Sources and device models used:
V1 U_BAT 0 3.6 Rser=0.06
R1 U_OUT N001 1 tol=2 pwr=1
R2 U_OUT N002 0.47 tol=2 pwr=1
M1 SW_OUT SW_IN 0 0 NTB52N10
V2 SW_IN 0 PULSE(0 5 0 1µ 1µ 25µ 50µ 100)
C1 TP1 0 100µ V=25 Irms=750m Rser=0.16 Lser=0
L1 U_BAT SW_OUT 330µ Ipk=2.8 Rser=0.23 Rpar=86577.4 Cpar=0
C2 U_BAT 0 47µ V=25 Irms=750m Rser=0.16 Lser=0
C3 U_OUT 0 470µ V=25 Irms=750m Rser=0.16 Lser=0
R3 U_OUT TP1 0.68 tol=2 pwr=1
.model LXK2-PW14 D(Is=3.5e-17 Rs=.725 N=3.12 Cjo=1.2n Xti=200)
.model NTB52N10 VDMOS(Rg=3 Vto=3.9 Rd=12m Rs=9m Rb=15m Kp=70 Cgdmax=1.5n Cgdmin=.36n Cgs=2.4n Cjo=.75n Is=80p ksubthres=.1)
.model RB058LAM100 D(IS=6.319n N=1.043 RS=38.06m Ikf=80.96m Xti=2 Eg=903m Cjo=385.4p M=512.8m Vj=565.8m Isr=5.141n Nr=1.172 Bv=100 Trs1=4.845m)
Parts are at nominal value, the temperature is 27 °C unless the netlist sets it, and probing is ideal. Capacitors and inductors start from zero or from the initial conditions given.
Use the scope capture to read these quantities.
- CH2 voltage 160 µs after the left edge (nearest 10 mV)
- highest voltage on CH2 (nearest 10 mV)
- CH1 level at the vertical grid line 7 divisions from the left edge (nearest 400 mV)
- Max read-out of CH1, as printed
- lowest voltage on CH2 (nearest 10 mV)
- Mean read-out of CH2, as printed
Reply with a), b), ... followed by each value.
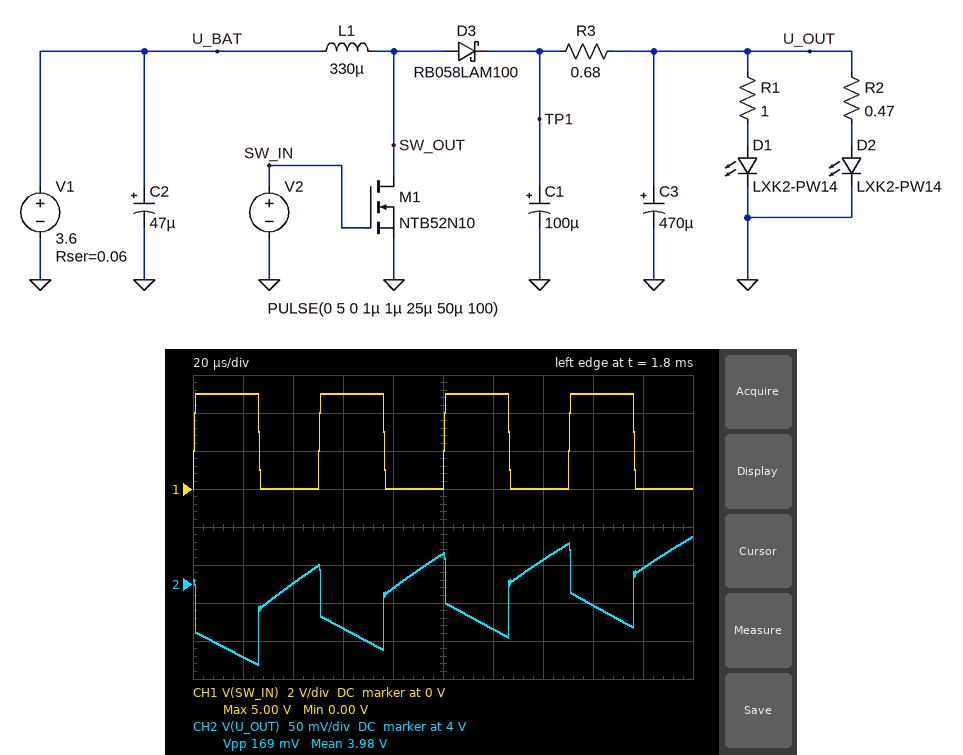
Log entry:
a) 3.97 V
b) 4.06 V
c) 0 V
d) 5.00 V
e) 3.89 V
f) 3.98 V
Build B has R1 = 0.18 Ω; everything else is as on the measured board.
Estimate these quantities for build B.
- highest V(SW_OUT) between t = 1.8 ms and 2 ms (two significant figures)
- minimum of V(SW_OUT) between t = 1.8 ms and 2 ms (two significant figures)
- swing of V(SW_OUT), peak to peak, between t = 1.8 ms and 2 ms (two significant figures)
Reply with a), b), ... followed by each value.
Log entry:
a) 6.0 V
b) 110 mV
c) 5.9 V
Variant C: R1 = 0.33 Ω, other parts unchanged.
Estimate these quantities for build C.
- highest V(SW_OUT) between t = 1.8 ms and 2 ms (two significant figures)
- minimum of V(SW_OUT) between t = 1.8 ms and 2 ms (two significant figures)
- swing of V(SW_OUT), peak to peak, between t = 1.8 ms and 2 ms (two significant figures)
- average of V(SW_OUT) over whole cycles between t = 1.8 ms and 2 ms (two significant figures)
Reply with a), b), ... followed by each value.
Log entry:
a) 6.0 V
b) 110 mV
c) 5.9 V
d) 3.0 V
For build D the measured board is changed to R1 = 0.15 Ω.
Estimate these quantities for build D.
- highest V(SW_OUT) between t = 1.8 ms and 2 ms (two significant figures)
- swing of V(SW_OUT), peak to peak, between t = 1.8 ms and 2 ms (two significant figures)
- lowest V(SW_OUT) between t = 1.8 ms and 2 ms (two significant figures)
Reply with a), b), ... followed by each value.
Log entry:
a) 6.0 V
b) 5.9 V
c) 110 mV
